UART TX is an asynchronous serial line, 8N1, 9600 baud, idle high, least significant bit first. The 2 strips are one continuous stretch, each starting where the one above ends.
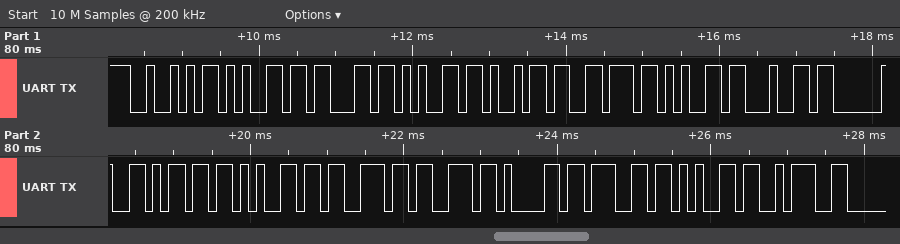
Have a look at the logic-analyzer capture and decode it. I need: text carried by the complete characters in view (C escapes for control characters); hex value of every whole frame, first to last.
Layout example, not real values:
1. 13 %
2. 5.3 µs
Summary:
1. "Received message:"
2. 52 65 63 65 69 76 65 64 20 6D 65 73 73 61 67 65 3A
